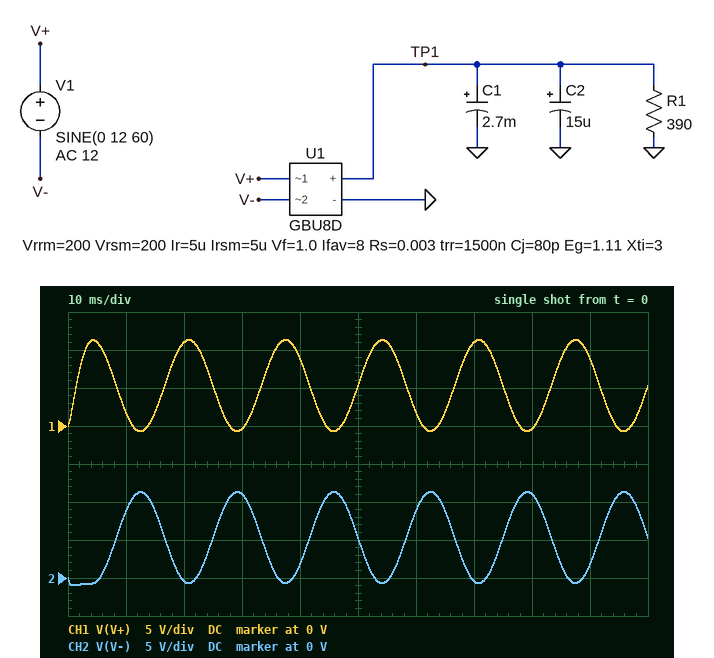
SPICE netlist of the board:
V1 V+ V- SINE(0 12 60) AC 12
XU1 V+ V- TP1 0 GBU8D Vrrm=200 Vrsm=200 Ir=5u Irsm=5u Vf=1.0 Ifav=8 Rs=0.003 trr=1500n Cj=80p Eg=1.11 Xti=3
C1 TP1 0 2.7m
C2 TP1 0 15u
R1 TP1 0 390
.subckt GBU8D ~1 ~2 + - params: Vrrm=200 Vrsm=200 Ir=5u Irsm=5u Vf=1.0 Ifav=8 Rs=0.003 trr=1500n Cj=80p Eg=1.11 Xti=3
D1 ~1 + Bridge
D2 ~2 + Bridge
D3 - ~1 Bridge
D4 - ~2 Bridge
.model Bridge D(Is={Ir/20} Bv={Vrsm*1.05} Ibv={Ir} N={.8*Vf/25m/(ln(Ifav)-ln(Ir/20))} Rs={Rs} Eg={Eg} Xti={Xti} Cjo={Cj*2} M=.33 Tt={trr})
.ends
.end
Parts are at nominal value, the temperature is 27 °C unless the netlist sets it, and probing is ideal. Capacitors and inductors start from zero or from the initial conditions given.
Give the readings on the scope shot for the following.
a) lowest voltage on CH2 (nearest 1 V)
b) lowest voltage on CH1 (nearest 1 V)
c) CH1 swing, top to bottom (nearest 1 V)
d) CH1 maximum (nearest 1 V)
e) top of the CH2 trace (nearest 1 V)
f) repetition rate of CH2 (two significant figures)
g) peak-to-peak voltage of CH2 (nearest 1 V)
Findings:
-1 V
-1 V
12 V
11 V
11 V
60 Hz
12 V
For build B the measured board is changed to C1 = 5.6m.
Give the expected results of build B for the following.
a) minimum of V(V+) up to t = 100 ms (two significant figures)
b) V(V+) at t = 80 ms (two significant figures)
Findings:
-720 mV
-380 mV
